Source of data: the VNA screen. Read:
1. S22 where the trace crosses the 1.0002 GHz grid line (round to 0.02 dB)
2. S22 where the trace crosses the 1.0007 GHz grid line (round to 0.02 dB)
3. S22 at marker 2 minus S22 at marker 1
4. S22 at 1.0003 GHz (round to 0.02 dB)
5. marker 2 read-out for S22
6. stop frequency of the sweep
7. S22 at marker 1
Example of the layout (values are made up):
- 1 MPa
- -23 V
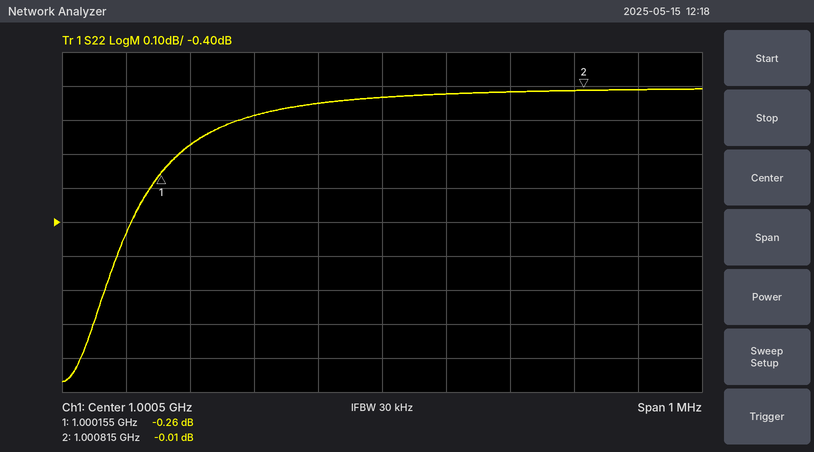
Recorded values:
- -0.18 dB
- -0.02 dB
- 0.25 dB
- -0.08 dB
- -0.01 dB
- 1.001 GHz
- -0.26 dB
